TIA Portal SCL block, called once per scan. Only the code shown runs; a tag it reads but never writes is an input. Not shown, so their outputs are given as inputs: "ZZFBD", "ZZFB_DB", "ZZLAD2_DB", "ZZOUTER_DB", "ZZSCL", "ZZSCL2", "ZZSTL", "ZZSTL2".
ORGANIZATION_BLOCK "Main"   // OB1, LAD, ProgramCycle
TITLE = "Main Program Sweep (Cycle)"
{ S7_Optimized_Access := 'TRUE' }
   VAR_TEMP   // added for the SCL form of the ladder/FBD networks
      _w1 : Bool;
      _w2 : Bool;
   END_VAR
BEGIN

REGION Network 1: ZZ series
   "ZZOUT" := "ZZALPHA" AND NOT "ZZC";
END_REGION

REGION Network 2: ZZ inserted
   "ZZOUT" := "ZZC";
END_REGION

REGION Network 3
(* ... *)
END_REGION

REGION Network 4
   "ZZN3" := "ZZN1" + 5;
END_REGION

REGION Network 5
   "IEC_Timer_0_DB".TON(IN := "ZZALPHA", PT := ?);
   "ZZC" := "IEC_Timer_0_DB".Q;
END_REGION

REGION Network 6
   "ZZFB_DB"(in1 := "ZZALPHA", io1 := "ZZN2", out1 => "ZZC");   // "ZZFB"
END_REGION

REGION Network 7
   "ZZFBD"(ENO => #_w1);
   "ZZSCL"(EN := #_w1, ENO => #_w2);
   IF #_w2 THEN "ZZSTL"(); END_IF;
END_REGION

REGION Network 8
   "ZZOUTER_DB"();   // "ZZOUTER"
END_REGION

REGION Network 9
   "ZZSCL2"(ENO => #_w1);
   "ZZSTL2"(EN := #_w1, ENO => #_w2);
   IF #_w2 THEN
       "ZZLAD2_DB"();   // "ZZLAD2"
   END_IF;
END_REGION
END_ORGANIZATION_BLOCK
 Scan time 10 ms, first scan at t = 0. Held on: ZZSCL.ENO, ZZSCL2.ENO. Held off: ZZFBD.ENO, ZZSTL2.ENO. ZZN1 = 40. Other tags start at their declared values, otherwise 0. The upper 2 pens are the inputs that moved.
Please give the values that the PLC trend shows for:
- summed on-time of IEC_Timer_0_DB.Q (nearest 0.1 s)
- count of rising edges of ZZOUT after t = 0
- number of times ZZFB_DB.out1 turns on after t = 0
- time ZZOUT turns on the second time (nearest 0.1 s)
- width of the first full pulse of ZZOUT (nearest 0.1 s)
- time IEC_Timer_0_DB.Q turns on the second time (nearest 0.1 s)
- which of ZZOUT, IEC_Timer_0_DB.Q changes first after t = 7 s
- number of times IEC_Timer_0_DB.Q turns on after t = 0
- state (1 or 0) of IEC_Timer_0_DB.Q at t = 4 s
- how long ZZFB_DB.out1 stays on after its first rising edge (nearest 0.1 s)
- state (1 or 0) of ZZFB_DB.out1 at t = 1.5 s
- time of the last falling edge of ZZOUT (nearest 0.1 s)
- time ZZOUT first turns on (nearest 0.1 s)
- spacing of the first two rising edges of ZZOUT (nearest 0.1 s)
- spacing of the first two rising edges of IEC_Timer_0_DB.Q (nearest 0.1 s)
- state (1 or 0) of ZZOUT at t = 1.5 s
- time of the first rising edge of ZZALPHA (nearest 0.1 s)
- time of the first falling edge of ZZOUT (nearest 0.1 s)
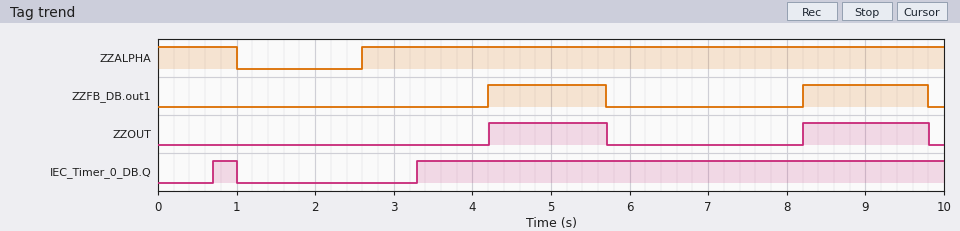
7.0 s
2
2
8.2 s
1.5 s
3.3 s
ZZOUT
2
1
1.5 s
0
9.8 s
4.2 s
4.0 s
2.6 s
0
2.6 s
5.7 s
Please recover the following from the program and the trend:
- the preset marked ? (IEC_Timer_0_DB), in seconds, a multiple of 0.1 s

0.7 s
